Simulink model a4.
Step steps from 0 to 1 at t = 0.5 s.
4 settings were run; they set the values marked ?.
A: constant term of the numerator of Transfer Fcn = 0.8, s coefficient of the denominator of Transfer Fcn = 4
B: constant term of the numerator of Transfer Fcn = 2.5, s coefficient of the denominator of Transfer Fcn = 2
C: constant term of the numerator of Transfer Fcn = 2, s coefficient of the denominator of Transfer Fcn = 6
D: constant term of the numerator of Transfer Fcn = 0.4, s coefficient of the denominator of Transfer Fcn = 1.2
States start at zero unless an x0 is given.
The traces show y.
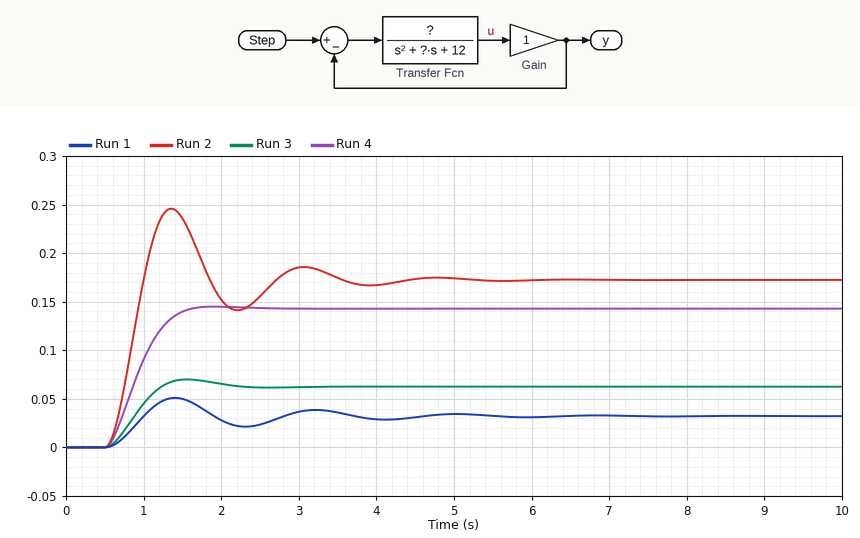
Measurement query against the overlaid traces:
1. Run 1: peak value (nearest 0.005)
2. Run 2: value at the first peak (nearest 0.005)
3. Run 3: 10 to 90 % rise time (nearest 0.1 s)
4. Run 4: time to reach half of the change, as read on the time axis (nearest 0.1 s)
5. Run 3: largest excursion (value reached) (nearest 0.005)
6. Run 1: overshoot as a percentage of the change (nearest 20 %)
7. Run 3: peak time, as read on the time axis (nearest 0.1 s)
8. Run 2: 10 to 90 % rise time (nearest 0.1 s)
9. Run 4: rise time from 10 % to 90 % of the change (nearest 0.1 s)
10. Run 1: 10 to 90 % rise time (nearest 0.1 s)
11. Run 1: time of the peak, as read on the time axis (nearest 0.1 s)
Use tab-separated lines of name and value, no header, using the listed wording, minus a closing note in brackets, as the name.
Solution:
Run 1: peak value	0.050
Run 2: value at the first peak	0.245
Run 3: 10 to 90 % rise time	0.5 s
Run 4: time to reach half of the change, as read on the time axis	0.9 s
Run 3: largest excursion (value reached)	0.070
Run 1: overshoot as a percentage of the change	60 %
Run 3: peak time, as read on the time axis	1.6 s
Run 2: 10 to 90 % rise time	0.3 s
Run 4: rise time from 10 % to 90 % of the change	0.7 s
Run 1: 10 to 90 % rise time	0.3 s
Run 1: time of the peak, as read on the time axis	1.4 s
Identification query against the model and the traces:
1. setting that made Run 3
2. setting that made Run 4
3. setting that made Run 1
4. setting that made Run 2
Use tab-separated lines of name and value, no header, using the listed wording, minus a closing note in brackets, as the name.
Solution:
setting that made Run 3	A
setting that made Run 4	C
setting that made Run 1	D
setting that made Run 2	B
